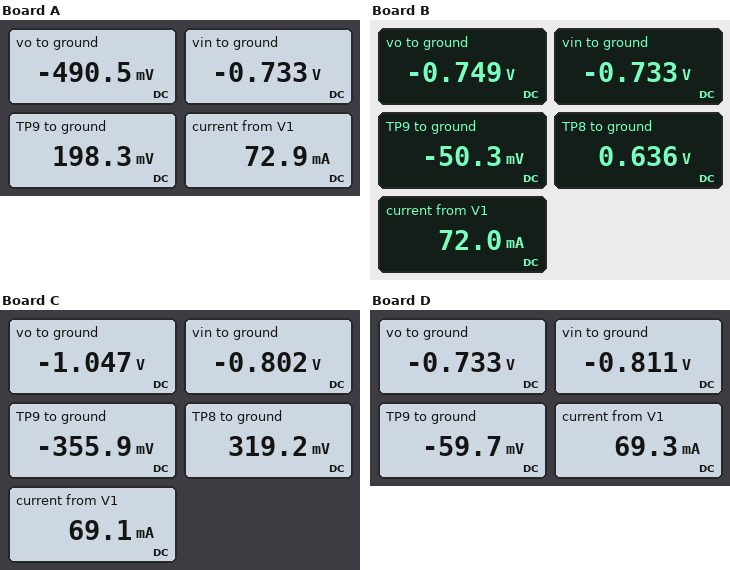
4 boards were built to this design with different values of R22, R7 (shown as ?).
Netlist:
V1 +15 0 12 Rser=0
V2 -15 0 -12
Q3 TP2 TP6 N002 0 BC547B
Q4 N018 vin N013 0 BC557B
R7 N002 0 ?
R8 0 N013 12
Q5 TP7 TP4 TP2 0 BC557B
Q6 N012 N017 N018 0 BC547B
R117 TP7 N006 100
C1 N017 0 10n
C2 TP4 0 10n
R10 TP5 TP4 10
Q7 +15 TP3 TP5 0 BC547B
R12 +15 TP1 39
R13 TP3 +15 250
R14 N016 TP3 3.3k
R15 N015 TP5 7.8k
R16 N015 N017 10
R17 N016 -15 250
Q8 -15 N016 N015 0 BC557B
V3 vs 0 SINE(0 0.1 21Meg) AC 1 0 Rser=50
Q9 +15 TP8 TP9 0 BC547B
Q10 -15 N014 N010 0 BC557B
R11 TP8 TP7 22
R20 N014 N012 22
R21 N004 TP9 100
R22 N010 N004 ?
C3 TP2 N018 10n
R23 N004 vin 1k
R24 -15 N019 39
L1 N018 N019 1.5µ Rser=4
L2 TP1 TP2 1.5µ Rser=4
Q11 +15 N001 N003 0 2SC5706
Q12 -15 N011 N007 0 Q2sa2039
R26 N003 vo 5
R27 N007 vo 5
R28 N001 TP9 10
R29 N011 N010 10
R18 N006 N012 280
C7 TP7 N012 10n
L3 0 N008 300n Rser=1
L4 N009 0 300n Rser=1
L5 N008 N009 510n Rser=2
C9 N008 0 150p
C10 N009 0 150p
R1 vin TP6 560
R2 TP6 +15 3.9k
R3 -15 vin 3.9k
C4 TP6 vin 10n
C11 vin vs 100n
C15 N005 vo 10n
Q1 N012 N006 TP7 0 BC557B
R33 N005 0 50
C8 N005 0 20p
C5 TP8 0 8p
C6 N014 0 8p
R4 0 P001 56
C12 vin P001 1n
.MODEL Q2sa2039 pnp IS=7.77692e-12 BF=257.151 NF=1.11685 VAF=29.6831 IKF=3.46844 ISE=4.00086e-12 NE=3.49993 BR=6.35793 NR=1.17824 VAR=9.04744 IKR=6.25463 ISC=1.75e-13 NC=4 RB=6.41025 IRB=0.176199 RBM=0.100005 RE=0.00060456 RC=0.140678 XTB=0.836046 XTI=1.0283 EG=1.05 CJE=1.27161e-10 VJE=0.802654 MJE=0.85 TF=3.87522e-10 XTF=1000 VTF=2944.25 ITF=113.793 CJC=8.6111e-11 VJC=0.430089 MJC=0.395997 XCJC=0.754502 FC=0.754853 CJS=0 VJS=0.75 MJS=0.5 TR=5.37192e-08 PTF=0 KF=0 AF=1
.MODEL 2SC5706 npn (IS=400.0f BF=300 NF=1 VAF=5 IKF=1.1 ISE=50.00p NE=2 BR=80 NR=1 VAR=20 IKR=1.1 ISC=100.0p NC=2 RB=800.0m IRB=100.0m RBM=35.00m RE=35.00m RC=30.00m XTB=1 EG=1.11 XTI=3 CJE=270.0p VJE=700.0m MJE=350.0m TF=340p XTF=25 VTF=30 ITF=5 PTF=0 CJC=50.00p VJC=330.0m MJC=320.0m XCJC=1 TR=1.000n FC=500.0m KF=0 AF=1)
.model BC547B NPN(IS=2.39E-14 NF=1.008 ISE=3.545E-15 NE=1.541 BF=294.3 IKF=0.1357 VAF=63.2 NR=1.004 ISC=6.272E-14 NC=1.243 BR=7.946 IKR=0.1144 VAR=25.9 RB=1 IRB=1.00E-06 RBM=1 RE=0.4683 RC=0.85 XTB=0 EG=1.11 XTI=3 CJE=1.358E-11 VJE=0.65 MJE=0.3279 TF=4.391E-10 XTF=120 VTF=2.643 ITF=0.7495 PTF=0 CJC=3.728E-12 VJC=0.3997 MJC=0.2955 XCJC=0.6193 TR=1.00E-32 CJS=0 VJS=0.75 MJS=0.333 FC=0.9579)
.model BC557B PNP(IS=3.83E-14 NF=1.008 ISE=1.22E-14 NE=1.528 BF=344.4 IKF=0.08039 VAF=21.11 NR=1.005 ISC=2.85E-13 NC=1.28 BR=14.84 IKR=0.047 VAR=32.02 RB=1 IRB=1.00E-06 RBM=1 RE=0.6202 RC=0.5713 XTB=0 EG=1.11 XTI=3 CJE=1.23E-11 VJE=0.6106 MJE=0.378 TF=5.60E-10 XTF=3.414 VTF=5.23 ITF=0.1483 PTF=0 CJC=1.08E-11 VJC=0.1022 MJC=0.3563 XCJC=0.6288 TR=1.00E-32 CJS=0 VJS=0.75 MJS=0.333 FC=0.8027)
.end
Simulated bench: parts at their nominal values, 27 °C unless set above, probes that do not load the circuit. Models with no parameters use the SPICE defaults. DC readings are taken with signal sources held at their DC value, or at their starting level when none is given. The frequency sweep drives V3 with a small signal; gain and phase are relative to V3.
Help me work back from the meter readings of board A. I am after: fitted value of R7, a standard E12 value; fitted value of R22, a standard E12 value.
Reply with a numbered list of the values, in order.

1. 27 Ω
2. 56 Ω
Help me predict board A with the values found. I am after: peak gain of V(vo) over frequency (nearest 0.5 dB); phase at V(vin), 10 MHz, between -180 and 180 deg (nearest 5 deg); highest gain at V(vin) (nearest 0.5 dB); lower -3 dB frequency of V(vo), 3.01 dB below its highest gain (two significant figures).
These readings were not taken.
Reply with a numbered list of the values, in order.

1. 26.0 dB
2. 55 deg
3. -4.0 dB
4. 31 kHz
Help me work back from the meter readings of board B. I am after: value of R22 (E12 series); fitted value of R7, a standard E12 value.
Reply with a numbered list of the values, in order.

1. 120 Ω
2. 27 Ω
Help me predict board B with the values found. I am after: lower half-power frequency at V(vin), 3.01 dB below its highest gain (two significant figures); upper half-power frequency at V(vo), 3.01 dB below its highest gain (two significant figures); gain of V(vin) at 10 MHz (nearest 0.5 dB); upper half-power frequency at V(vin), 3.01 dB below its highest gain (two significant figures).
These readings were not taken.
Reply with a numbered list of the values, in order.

1. 12 MHz
2. 21 MHz
3. -8.5 dB
4. 60 MHz
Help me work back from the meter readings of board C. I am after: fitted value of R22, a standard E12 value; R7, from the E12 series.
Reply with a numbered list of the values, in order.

1. 220 Ω
2. 8.2 Ω
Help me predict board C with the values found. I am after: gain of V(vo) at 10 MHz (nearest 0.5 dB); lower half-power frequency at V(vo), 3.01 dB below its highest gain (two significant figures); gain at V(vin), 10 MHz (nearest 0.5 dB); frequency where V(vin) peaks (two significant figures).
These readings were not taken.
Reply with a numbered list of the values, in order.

1. 27.0 dB
2. 47 kHz
3. -12.0 dB
4. 28 MHz
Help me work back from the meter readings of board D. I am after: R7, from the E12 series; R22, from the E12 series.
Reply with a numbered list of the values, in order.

1. 6.8 Ω
2. 82 Ω
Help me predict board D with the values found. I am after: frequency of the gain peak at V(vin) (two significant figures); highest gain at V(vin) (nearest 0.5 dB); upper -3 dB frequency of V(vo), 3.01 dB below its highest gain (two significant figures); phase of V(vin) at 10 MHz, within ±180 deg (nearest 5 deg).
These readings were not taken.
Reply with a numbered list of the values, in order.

1. 30 MHz
2. -2.5 dB
3. 34 MHz
4. 75 deg
